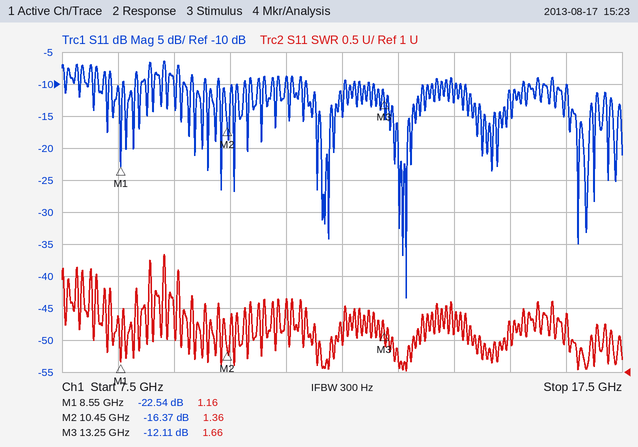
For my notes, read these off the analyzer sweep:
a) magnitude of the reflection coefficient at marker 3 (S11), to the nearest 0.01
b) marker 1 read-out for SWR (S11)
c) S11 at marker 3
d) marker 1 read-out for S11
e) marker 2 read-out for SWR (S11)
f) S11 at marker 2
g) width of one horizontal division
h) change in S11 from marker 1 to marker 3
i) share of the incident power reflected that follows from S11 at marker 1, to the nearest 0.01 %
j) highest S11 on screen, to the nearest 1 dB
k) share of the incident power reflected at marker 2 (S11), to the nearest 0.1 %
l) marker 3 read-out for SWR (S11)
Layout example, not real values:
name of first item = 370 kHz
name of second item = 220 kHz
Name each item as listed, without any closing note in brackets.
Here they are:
magnitude of the reflection coefficient at marker 3 (S11), to the nearest 0.01 = 0.25
marker 1 read-out for SWR = 1.16
S11 at marker 3 = -12.11 dB
marker 1 read-out for S11 = -22.54 dB
marker 2 read-out for SWR = 1.36
S11 at marker 2 = -16.37 dB
width of one horizontal division = 1 GHz
change in S11 from marker 1 to marker 3 = 10.43 dB
share of the incident power reflected that follows from S11 at marker 1, to the nearest 0.01 % = 0.56 %
highest S11 on screen, to the nearest 1 dB = -6 dB
share of the incident power reflected at marker 2 (S11), to the nearest 0.1 % = 2.3 %
marker 3 read-out for SWR = 1.66
